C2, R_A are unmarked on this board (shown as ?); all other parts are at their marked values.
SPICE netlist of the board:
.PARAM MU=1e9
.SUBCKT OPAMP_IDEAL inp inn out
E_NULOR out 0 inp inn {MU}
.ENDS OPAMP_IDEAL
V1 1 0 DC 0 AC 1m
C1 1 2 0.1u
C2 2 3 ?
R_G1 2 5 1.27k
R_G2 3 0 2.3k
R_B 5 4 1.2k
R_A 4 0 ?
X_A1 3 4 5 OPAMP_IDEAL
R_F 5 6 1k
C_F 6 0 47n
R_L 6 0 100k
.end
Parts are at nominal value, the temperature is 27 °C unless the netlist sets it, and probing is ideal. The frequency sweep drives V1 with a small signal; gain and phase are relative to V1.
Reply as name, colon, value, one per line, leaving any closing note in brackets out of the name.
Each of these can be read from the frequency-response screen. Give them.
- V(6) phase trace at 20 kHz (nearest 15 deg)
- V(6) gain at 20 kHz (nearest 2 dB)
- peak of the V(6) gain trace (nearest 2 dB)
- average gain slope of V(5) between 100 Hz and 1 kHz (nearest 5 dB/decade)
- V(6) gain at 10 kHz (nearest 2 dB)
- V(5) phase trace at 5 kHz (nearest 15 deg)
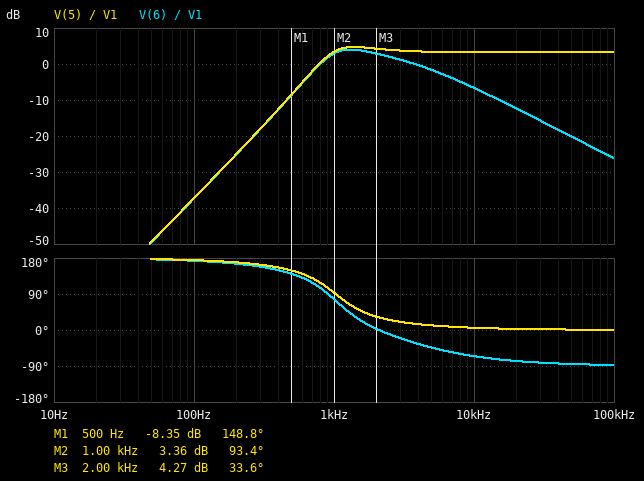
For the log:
V(6) phase trace at 20 kHz: -75 deg
V(6) gain at 20 kHz: -12 dB
peak of the V(6) gain trace: 4 dB
average gain slope of V(5) between 100 Hz and 1 kHz: 40 dB/decade
V(6) gain at 10 kHz: -6 dB
V(5) phase trace at 5 kHz: 15 deg
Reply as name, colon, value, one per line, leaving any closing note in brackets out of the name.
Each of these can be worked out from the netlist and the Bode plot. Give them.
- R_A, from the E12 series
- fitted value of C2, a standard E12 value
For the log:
R_A, from the E12 series: 2.7 kΩ
fitted value of C2, a standard E12 value: 82 nF
